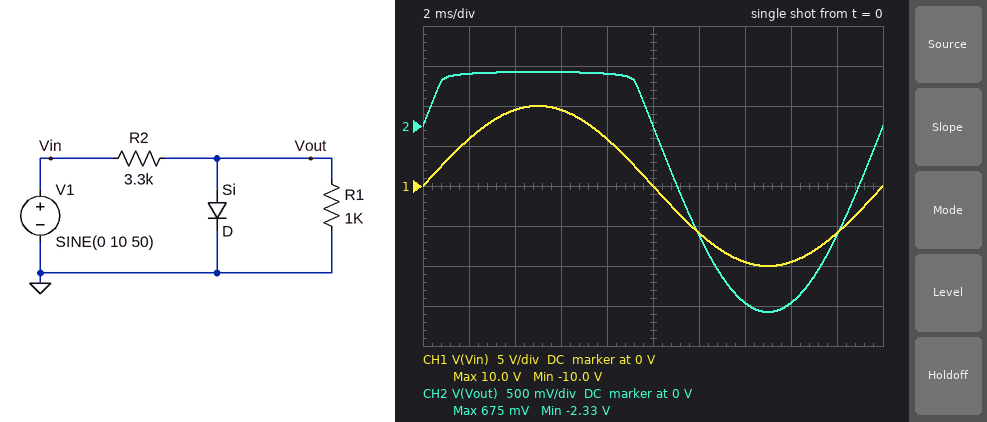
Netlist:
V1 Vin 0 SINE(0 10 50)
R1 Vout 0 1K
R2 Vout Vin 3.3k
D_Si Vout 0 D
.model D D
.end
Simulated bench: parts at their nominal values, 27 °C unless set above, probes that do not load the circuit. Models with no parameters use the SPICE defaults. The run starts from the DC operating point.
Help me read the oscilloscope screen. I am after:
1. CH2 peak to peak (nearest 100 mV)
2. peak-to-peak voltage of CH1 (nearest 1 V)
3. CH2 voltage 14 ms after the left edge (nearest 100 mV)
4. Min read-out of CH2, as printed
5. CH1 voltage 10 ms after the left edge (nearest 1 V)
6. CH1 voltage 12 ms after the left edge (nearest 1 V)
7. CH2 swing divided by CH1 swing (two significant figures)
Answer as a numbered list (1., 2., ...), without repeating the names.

1. 3.0 V
2. 20 V
3. -2.2 V
4. -2.33 V
5. 0 V
6. -6 V
7. 0.15
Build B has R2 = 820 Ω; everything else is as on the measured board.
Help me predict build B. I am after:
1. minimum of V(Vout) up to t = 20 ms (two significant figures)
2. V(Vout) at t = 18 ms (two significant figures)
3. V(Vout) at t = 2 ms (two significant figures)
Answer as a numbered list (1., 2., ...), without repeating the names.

1. -5.5 V
2. -3.2 V
3. 700 mV
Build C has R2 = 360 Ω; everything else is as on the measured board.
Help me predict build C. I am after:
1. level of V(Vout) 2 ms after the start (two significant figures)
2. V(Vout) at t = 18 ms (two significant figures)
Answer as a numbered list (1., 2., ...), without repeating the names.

1. 720 mV
2. -4.3 V
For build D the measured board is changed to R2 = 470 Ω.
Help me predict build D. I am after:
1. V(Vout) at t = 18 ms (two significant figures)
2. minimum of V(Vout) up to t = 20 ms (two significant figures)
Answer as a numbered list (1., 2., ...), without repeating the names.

1. -4.0 V
2. -6.8 V
